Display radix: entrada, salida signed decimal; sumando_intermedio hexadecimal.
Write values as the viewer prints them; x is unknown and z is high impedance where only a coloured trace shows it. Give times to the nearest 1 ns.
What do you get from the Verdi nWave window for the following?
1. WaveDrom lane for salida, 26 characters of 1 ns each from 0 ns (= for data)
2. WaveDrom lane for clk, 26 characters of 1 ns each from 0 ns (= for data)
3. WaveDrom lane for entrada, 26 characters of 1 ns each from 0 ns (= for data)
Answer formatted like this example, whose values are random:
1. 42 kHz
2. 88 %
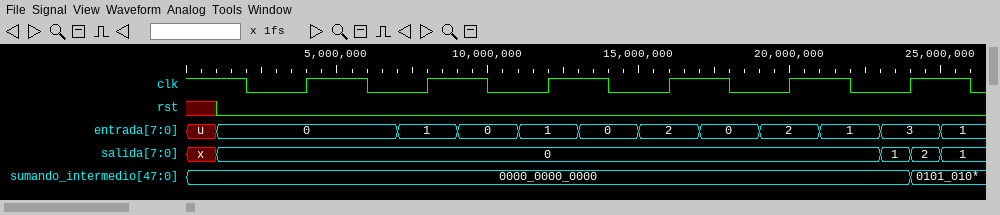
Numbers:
1. {name: 'salida', wave: 'x=.....................===', data: '0 1 2 1'}
2. {name: 'clk', wave: '1.0.1.0.1.0.1.0.1.0.1.0.1.'}
3. {name: 'entrada', wave: 'x=.....=.=.=.=.=.=.=.=.=.=', data: '0 1 0 1 0 2 0 2 1 3 1'}
